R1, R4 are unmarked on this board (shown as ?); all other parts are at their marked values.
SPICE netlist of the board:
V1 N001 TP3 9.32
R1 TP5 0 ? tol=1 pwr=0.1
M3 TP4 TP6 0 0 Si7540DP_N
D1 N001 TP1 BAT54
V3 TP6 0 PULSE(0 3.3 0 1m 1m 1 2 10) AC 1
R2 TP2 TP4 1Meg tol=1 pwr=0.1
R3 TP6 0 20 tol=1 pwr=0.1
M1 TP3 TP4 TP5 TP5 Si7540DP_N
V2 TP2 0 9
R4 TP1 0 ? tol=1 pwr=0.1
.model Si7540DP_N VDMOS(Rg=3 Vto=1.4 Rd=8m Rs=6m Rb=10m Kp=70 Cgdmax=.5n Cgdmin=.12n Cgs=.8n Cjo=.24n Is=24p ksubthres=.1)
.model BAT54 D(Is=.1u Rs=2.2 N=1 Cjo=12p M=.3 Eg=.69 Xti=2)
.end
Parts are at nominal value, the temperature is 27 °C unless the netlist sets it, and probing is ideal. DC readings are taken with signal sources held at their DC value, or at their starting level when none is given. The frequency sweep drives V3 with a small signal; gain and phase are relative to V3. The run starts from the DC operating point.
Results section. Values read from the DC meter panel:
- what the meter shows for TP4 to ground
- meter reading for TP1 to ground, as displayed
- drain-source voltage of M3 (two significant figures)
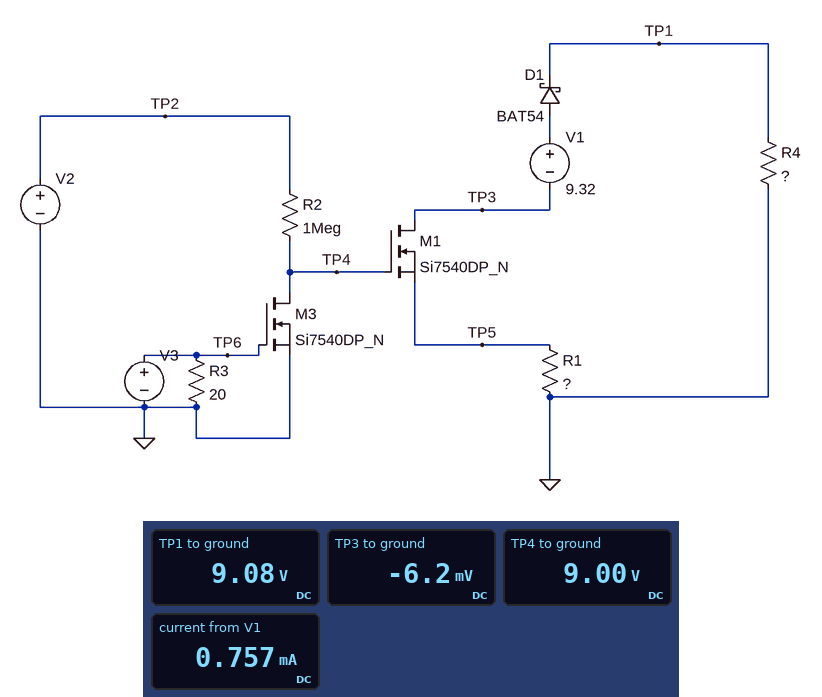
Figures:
9.00 V
9.08 V
9.0 V
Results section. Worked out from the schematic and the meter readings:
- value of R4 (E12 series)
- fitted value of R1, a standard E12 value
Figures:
12 kΩ
8.2 Ω
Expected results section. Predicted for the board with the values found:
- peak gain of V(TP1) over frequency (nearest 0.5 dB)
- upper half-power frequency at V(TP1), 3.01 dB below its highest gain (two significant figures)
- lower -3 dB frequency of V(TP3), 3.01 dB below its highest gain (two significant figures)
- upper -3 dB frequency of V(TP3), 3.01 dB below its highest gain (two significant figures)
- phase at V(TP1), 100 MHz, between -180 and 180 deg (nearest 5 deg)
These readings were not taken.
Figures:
-14.0 dB
180 MHz
28 MHz
180 MHz
-20 deg
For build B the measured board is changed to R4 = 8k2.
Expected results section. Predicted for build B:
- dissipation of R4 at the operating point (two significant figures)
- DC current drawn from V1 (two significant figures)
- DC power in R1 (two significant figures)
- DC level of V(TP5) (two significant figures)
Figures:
10 mW
1.1 mA
10 µW
-9.1 mV
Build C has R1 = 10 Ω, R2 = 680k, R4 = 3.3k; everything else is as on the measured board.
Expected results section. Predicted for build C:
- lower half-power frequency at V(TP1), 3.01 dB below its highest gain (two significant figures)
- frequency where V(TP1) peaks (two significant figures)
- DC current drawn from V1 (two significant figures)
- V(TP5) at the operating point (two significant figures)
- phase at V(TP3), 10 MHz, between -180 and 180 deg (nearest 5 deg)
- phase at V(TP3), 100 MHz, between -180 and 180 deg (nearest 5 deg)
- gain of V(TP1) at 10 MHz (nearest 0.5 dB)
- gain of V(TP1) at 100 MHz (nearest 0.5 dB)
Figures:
26 MHz
66 MHz
2.7 mA
-27 mV
70 deg
-20 deg
-23.0 dB
-13.5 dB
